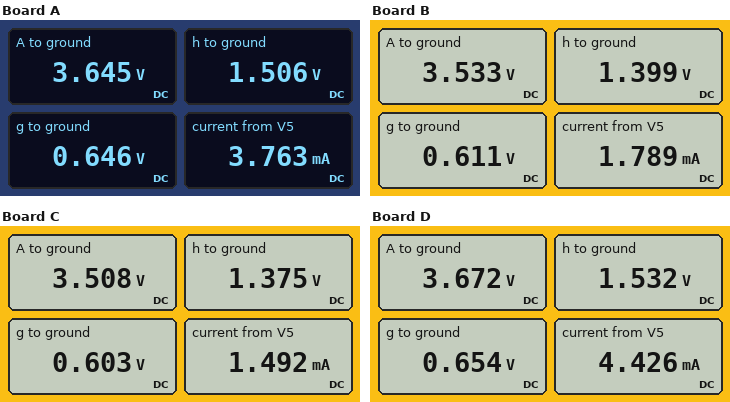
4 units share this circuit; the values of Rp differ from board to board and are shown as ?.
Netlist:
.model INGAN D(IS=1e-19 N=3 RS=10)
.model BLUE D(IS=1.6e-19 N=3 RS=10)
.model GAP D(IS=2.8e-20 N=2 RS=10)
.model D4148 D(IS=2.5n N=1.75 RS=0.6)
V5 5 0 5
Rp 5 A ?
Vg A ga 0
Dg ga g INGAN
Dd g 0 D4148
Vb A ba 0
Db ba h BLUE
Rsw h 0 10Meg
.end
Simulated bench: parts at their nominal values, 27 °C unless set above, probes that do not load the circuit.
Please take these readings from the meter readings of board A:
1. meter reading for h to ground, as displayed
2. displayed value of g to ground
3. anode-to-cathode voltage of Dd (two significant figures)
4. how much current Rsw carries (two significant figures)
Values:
1.506 V
0.646 V
650 mV
150 nA
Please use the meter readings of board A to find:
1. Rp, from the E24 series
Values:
360 Ω
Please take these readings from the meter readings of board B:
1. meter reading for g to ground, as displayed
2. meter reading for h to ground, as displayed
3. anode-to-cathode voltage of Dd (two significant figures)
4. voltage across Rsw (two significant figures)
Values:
0.611 V
1.399 V
610 mV
1.4 V
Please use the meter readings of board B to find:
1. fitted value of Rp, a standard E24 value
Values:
820 Ω
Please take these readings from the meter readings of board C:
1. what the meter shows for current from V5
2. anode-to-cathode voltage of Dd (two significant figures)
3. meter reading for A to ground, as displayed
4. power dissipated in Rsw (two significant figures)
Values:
1.492 mA
600 mV
3.508 V
190 nW
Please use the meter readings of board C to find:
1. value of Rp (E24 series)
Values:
1 kΩ
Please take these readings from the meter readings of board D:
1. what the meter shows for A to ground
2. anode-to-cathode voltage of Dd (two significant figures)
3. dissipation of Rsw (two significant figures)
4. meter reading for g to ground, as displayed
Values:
3.672 V
650 mV
230 nW
0.654 V
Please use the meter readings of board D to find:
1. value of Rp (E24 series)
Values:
300 Ω
